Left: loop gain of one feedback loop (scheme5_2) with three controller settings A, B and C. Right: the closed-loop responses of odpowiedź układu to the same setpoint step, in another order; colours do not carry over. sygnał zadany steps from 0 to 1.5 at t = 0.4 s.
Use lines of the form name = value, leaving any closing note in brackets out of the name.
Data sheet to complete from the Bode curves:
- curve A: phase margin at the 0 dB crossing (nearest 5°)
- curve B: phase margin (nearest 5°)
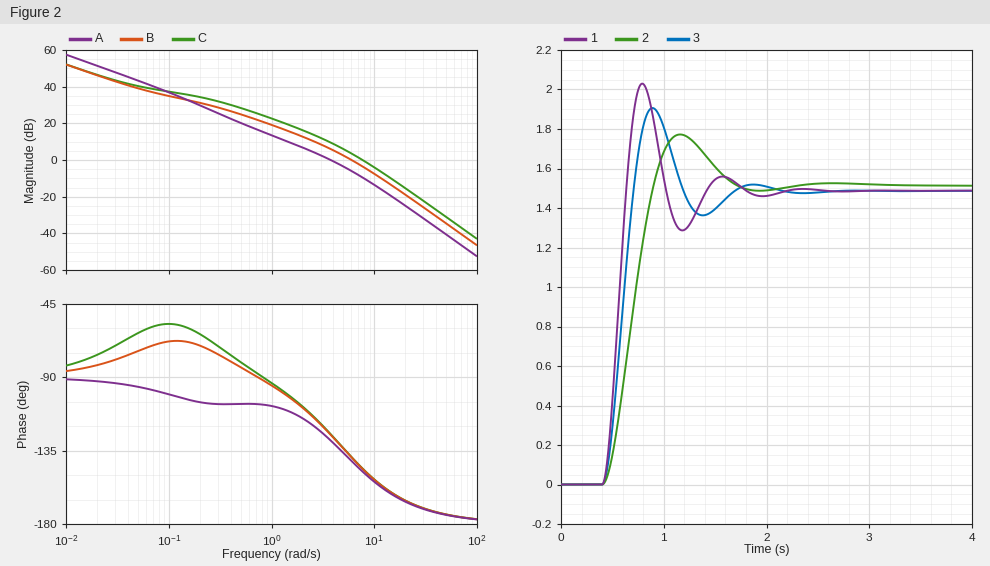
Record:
curve A: phase margin at the 0 dB crossing = 50°
curve B: phase margin = 40°
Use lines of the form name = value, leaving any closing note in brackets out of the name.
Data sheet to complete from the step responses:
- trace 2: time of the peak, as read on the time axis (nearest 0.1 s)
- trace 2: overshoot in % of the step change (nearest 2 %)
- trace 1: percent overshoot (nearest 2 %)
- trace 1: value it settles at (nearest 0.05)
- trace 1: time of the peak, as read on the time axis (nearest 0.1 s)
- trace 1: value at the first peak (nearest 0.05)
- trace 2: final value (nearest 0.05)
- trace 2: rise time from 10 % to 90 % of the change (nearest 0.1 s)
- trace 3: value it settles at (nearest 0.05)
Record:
trace 2: time of the peak, as read on the time axis = 1.2 s
trace 2: overshoot in % of the step change = 18 %
trace 1: percent overshoot = 36 %
trace 1: value it settles at = 1.50
trace 1: time of the peak, as read on the time axis = 0.8 s
trace 1: value at the first peak = 2.05
trace 2: final value = 1.50
trace 2: rise time from 10 % to 90 % of the change = 0.3 s
trace 3: value it settles at = 1.50
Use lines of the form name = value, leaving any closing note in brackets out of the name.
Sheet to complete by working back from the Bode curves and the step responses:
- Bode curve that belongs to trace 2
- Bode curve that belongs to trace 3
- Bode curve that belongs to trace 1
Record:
Bode curve that belongs to trace 2 = A
Bode curve that belongs to trace 3 = B
Bode curve that belongs to trace 1 = C
